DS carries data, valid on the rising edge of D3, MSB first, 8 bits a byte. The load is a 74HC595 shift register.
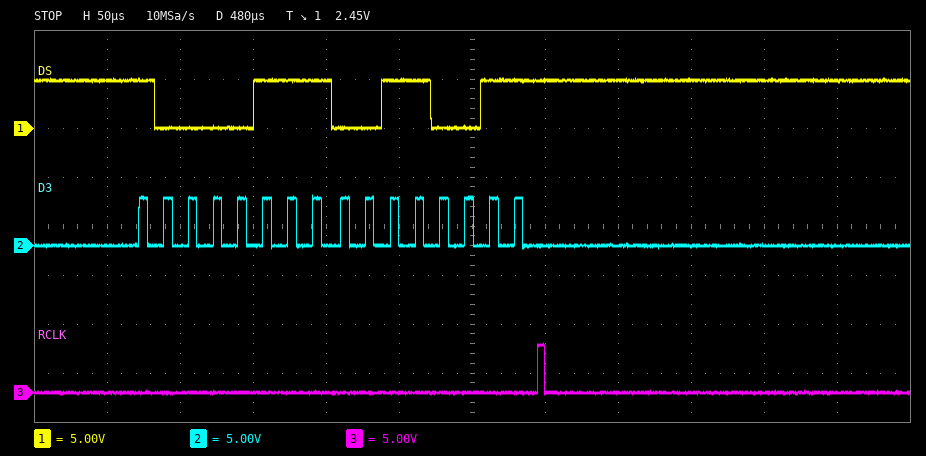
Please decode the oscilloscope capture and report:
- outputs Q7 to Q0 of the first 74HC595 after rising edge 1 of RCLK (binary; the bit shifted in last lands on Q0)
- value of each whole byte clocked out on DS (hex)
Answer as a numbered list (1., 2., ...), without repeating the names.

1. 00110011
2. 87 33
